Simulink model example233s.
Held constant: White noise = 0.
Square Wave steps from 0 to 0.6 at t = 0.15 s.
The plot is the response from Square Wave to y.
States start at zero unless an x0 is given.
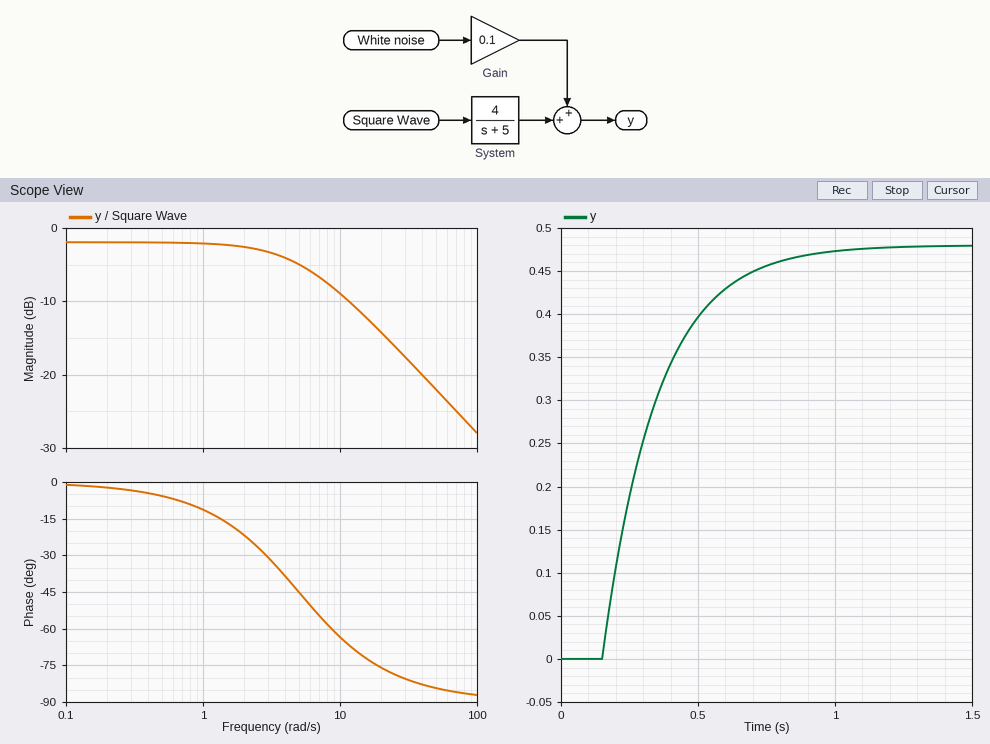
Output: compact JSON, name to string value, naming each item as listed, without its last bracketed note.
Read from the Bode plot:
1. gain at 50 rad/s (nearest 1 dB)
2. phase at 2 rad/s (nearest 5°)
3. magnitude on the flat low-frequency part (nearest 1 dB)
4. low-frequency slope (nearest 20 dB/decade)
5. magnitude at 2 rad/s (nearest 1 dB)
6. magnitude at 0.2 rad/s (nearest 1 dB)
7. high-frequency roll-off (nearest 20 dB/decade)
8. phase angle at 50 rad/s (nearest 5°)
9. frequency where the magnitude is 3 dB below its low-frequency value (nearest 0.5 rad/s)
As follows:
{"gain at 50 rad/s": "-22 dB", "phase at 2 rad/s": "-20°", "magnitude on the flat low-frequency part": "-2 dB", "low-frequency slope": "0 dB/decade", "magnitude at 2 rad/s": "-3 dB", "magnitude at 0.2 rad/s": "-2 dB", "high-frequency roll-off": "-20 dB/decade", "phase angle at 50 rad/s": "-85°", "frequency where the magnitude is 3 dB below its low-frequency value": "5.0 rad/s"}
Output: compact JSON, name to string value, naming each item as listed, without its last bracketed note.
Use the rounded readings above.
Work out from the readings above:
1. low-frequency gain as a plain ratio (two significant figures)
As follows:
{"low-frequency gain as a plain ratio": "0.79"}
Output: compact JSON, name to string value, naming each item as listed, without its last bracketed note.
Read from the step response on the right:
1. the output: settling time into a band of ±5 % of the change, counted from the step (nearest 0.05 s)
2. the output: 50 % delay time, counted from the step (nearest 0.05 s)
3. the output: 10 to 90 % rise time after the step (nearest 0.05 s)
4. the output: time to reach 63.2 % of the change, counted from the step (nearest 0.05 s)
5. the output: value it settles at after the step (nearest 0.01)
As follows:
{"the output: settling time into a band of ±5 % of the change, counted from the step": "0.60 s", "the output: 50 % delay time, counted from the step": "0.15 s", "the output: 10 to 90 % rise time after the step": "0.45 s", "the output: time to reach 63.2 % of the change, counted from the step": "0.20 s", "the output: value it settles at after the step": "0.48"}
